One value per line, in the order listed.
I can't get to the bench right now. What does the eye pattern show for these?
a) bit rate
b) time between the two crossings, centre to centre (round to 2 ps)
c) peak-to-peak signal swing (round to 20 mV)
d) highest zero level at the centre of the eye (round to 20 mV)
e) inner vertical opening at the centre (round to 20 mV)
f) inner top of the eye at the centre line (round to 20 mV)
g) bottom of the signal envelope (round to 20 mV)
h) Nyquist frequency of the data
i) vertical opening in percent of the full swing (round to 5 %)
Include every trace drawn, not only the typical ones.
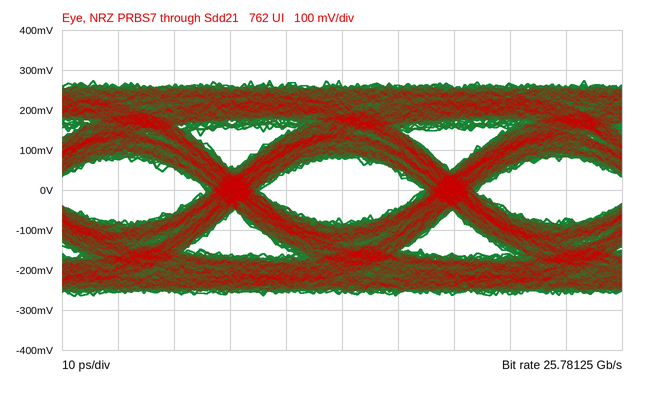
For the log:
25.78125 Gb/s
38 ps
540 mV
-80 mV
160 mV
80 mV
-260 mV
12.89062 GHz
30 %
